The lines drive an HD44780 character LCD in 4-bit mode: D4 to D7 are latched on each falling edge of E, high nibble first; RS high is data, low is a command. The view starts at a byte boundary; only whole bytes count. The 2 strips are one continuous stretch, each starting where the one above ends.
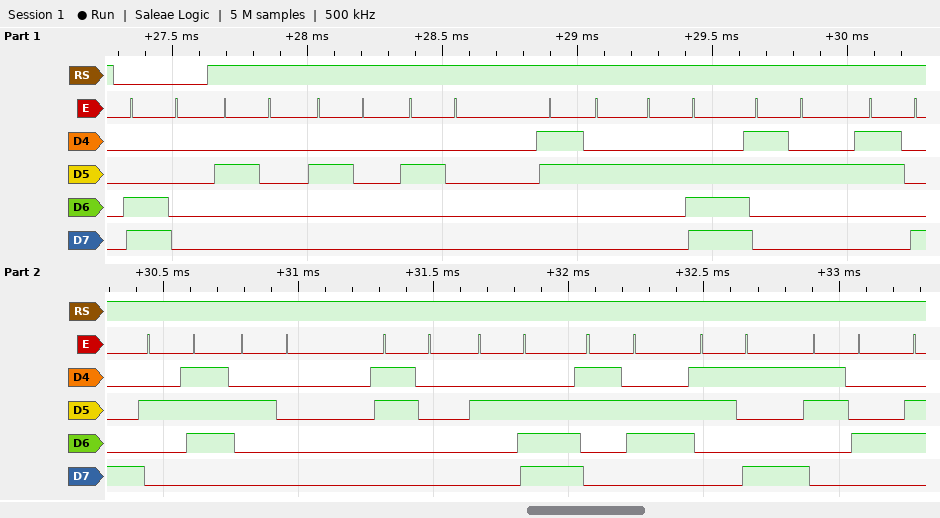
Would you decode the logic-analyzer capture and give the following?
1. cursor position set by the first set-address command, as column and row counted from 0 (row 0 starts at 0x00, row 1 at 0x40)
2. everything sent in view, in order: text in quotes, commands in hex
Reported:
column 0, row 1
0xC0 "   2.28' 0.694"
